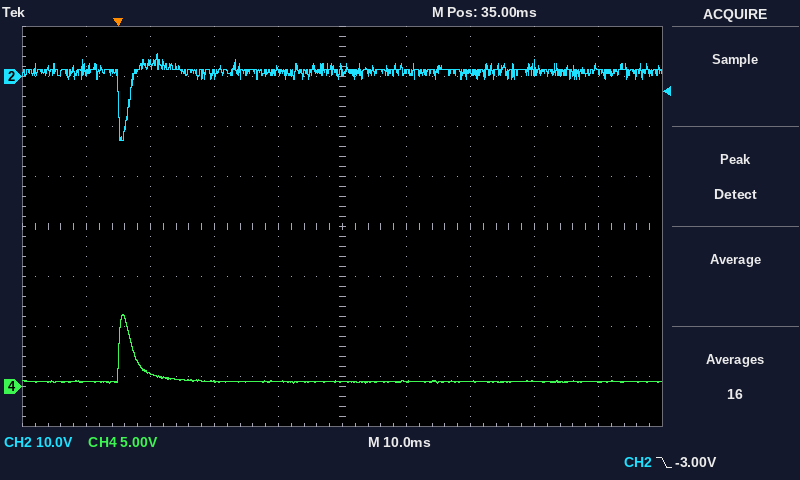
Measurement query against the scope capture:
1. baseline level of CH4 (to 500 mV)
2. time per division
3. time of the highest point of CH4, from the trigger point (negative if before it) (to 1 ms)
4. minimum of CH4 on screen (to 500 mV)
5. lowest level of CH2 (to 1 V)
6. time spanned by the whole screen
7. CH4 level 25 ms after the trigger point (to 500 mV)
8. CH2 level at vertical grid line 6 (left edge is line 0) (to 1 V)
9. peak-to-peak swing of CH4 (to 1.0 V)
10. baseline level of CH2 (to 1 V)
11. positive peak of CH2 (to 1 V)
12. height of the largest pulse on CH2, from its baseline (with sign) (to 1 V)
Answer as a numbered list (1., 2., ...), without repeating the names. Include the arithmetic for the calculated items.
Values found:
1. 500 mV
2. 10 ms
3. +1 ms
4. 500 mV
5. -13 V
6. 100 ms
7. 500 mV
8. 1 V
9. 7.0 V
10. 1 V
11. 5 V
12. -13 V − (1 V) = -14 V
